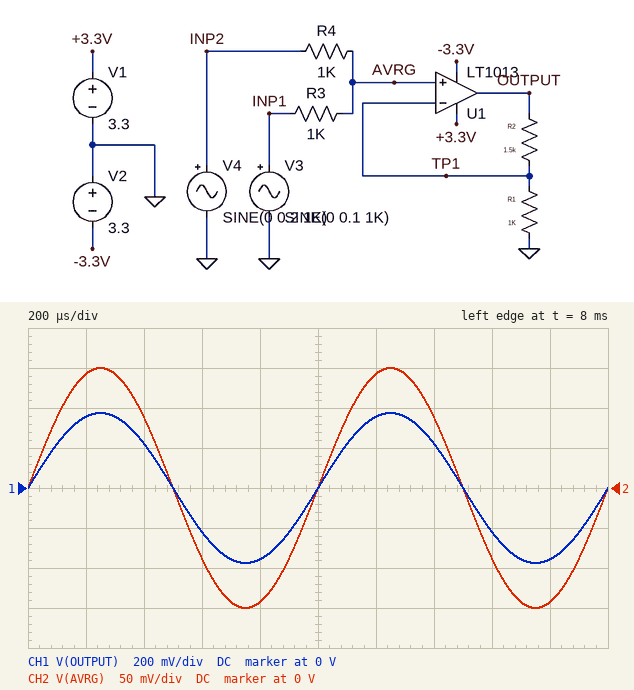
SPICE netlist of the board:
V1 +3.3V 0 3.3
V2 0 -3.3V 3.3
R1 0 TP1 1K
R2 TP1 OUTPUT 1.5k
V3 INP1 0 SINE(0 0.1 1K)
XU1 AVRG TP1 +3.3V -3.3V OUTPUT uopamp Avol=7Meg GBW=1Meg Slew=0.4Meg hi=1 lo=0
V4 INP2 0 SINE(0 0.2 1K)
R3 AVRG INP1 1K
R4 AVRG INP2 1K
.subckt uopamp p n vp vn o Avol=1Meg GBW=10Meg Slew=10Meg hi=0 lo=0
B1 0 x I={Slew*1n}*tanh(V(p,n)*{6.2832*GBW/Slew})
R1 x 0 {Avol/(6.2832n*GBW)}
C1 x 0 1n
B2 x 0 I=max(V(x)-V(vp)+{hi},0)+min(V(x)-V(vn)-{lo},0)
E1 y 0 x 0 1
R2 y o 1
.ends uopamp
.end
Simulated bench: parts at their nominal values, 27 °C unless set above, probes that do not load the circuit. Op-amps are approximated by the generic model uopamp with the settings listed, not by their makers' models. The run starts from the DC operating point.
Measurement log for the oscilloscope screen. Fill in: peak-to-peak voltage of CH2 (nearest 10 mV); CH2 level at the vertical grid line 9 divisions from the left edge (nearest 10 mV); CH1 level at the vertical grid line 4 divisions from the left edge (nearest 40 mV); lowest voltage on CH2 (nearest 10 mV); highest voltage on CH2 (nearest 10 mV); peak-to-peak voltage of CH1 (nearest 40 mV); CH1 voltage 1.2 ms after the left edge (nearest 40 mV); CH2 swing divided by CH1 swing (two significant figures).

300 mV
-140 mV
-360 mV
-150 mV
150 mV
760 mV
360 mV
0.40
